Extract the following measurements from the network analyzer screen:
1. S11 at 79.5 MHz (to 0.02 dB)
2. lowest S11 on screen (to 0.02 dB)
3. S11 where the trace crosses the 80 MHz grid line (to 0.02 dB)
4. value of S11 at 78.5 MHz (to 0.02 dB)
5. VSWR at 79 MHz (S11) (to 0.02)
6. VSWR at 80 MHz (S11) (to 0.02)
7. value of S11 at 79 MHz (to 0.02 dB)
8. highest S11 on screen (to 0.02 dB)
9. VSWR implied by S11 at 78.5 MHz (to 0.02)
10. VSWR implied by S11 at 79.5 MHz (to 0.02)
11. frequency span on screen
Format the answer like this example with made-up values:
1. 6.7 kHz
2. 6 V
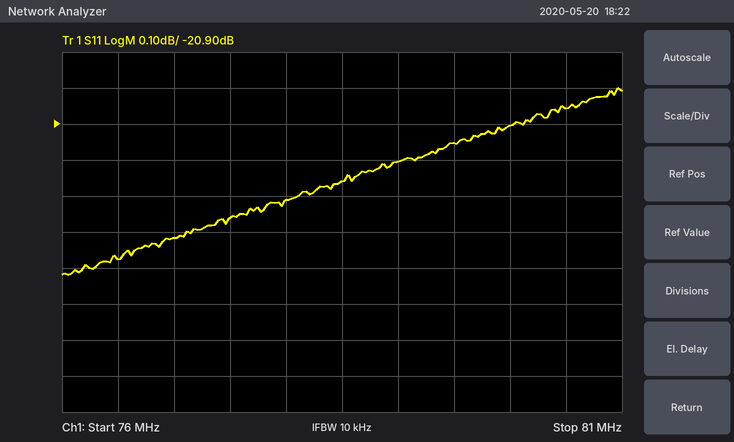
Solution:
1. -20.96 dB
2. -21.32 dB
3. -20.90 dB
4. -21.06 dB
5. 1.20
6. 1.20
7. -21.00 dB
8. -20.80 dB
9. 1.20
10. 1.20
11. 5 MHz
